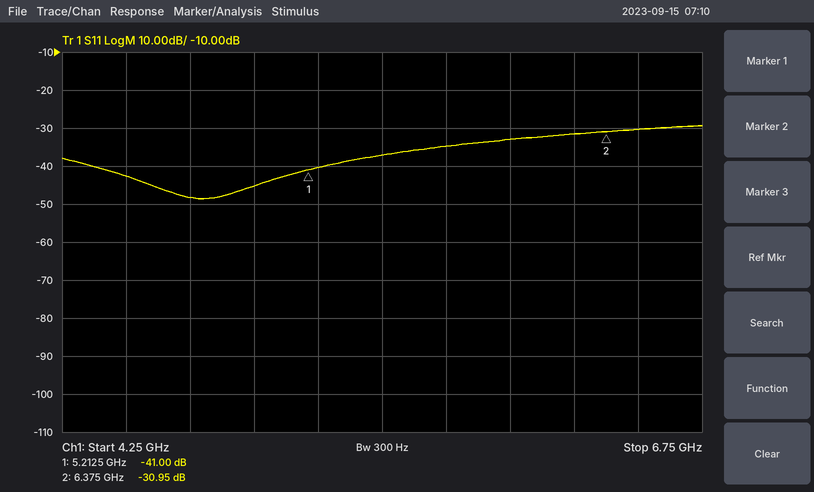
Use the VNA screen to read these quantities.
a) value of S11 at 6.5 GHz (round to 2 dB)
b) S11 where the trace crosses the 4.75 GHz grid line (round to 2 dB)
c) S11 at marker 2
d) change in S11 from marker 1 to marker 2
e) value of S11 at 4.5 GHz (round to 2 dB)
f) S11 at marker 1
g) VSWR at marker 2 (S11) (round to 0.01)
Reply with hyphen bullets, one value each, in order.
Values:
- -30 dB
- -48 dB
- -30.95 dB
- 10.05 dB
- -42 dB
- -41.00 dB
- 1.06
